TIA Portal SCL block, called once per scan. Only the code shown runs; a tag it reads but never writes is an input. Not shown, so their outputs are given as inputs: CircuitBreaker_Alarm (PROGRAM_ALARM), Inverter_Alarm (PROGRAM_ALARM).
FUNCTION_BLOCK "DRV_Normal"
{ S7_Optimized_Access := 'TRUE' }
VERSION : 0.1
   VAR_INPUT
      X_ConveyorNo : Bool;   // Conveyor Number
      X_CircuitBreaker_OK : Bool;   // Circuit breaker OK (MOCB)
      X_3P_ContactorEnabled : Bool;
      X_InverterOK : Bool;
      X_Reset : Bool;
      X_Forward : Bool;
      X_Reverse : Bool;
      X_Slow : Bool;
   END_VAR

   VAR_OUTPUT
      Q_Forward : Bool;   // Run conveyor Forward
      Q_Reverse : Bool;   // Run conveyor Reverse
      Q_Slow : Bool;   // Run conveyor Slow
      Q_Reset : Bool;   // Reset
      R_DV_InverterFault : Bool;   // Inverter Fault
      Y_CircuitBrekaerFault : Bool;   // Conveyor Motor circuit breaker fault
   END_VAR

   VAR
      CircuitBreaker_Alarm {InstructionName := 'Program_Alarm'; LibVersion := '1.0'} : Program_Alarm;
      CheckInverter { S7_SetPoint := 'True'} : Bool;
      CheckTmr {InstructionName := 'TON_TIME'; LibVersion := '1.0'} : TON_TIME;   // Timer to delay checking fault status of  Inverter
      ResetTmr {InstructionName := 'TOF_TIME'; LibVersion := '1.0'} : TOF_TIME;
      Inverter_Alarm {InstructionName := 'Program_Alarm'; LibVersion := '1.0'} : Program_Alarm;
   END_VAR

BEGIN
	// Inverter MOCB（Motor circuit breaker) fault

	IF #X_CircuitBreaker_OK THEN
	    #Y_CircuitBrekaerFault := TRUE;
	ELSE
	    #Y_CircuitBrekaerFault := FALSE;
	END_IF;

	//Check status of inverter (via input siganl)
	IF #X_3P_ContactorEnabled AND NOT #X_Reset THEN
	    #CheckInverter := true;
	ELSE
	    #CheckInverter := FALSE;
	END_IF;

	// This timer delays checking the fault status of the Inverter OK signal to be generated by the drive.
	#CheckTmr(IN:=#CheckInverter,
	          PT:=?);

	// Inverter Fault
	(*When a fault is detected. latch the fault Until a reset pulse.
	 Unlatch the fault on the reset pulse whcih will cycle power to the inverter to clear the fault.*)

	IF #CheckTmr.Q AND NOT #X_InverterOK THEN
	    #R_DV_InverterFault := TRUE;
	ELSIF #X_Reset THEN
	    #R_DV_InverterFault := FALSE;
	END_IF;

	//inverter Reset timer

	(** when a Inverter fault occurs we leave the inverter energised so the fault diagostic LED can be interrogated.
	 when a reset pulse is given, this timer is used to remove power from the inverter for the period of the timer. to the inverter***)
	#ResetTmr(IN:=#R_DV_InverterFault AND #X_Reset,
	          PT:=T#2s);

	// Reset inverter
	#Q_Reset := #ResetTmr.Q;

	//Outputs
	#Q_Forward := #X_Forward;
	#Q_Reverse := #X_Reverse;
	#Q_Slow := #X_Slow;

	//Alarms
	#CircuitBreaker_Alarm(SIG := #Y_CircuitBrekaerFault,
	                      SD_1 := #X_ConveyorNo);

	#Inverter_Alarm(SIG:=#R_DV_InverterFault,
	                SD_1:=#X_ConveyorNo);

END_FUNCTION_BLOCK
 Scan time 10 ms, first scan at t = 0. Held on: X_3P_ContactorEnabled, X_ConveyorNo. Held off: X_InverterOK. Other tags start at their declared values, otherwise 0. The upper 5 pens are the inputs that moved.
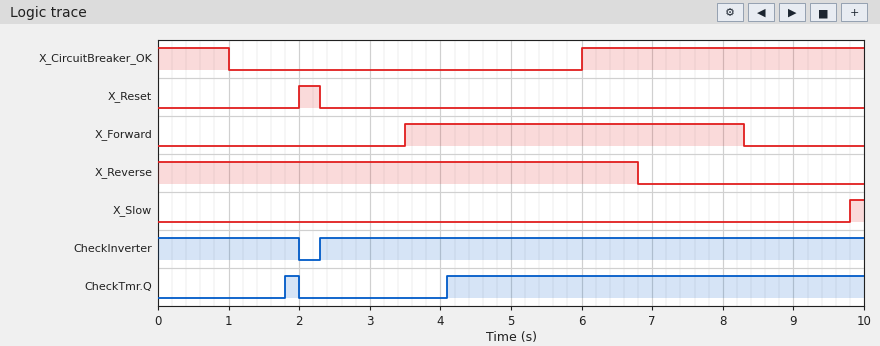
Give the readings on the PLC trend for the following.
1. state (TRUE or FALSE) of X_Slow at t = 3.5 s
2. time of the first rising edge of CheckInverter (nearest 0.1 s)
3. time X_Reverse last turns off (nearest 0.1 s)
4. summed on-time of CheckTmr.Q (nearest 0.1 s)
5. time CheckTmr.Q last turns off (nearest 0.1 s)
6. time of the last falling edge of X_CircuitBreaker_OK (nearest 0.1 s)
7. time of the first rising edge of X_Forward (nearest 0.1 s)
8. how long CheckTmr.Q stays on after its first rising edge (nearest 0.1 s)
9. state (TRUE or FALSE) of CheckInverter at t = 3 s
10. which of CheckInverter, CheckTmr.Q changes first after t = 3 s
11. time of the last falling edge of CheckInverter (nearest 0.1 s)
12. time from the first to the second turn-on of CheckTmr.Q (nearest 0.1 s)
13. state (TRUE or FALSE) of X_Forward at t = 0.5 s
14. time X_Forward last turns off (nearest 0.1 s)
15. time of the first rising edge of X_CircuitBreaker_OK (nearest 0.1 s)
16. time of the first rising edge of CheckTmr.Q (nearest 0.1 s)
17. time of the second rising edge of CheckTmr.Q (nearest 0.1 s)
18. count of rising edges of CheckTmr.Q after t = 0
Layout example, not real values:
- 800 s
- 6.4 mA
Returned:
- FALSE
- 2.3 s
- 6.8 s
- 6.1 s
- 2.0 s
- 1.0 s
- 3.5 s
- 0.2 s
- TRUE
- CheckTmr.Q
- 2.0 s
- 2.3 s
- FALSE
- 8.3 s
- 6.0 s
- 1.8 s
- 4.1 s
- 2
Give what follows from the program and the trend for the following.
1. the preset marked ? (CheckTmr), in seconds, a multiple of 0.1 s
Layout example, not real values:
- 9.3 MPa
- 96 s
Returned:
- 1.8 s
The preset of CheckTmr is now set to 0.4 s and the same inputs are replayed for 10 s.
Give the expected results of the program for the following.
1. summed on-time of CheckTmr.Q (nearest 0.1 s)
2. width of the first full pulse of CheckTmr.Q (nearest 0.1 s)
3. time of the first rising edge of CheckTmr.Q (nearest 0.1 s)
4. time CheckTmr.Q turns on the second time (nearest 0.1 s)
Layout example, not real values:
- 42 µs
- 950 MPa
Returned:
- 8.9 s
- 1.6 s
- 0.4 s
- 2.7 s
